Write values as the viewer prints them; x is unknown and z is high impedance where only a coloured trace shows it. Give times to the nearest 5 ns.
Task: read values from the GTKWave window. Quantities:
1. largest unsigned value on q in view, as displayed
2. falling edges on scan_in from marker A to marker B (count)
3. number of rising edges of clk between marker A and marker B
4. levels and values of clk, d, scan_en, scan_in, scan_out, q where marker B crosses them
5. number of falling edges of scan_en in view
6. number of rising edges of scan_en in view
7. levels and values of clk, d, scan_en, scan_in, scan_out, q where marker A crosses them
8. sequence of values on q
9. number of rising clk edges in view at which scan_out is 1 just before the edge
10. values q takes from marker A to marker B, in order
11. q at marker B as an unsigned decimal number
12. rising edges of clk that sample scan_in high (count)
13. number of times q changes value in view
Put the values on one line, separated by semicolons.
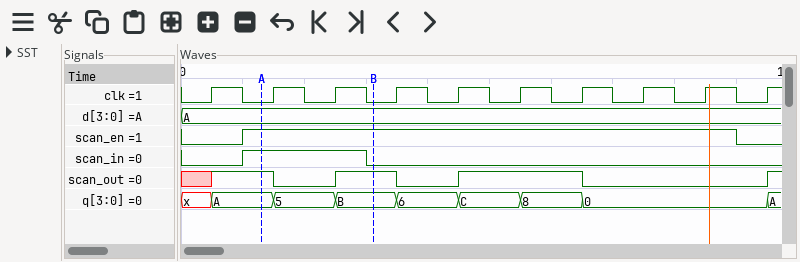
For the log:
C; 1; 2; clk=0, d=A, scan_en=1, scan_in=0, scan_out=1, q=B; 1; 1; clk=0, d=A, scan_en=1, scan_in=1, scan_out=1, q=A; x, A, 5, B, 6, C, 8, 0, A; 4; A, 5, B; 11; 2; 8
